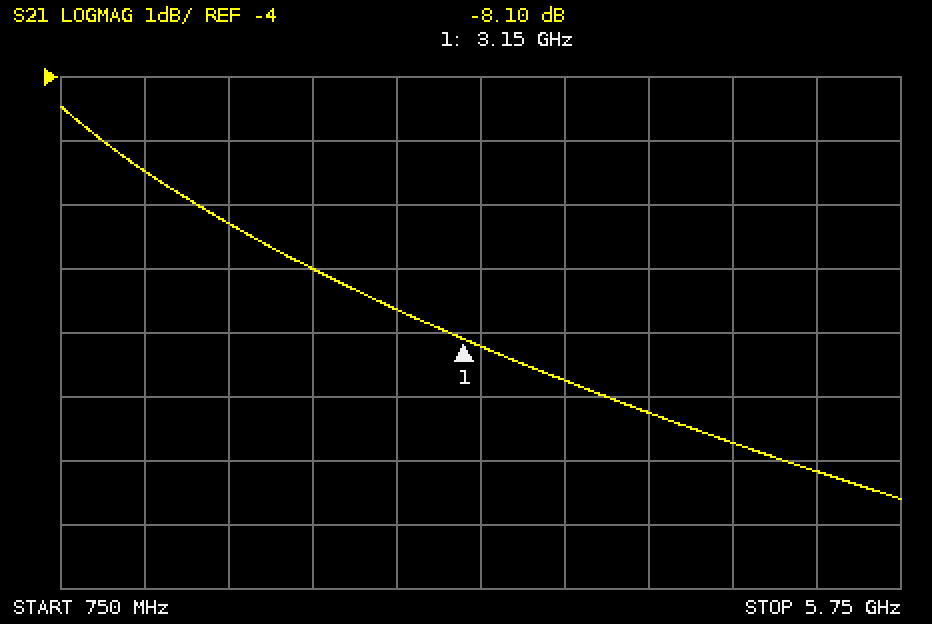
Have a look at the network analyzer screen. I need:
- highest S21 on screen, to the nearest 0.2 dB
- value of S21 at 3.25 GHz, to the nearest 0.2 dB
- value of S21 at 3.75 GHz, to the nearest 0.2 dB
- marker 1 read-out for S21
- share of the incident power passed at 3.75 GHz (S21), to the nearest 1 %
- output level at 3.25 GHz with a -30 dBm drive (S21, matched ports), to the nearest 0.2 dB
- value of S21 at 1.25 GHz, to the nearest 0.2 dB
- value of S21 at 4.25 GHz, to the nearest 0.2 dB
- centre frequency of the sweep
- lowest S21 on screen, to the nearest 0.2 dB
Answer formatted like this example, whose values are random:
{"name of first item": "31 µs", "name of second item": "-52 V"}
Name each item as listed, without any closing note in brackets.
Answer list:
{"highest S21 on screen, to the nearest 0.2 dB": "-4.4 dB", "value of S21 at 3.25 GHz, to the nearest 0.2 dB": "-8.2 dB", "value of S21 at 3.75 GHz, to the nearest 0.2 dB": "-8.8 dB", "marker 1 read-out for S21": "-8.10 dB", "share of the incident power passed at 3.75 GHz (S21), to the nearest 1 %": "13 %", "output level at 3.25 GHz with a -30 dBm drive (S21, matched ports), to the nearest 0.2 dB": "-38.2 dBm", "value of S21 at 1.25 GHz, to the nearest 0.2 dB": "-5.4 dB", "value of S21 at 4.25 GHz, to the nearest 0.2 dB": "-9.2 dB", "centre frequency of the sweep": "3.25 GHz", "lowest S21 on screen, to the nearest 0.2 dB": "-10.6 dB"}
